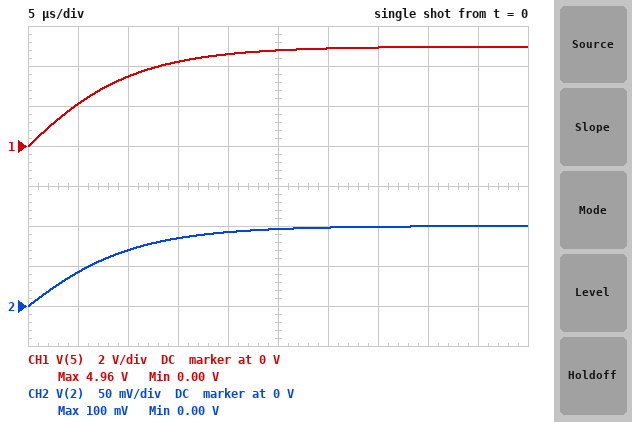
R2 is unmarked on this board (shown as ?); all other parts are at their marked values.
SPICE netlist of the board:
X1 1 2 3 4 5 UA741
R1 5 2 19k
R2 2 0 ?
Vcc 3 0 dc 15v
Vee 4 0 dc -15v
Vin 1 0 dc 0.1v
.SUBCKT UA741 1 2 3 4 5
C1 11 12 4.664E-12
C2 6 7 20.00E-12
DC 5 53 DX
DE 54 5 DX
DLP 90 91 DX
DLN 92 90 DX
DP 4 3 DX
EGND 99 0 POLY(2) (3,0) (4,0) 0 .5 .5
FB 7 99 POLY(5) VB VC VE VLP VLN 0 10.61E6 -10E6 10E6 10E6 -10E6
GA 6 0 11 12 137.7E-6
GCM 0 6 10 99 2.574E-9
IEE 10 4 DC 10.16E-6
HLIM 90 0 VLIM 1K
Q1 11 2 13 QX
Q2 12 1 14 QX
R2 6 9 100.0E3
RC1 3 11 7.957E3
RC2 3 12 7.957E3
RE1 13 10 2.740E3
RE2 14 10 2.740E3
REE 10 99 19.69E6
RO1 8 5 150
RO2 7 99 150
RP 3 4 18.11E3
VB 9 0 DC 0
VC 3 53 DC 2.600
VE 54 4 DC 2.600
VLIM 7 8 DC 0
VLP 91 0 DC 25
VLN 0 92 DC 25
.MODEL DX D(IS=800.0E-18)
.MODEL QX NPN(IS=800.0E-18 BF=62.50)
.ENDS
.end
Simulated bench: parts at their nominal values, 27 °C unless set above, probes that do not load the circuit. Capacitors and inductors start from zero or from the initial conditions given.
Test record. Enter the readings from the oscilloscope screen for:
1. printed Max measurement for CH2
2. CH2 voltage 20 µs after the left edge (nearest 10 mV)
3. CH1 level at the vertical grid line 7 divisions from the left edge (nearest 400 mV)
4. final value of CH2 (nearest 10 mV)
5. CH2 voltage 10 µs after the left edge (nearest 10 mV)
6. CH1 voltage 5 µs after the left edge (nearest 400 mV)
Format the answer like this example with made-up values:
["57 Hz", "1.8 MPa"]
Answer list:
["100 mV", "90 mV", "4.8 V", "100 mV", "70 mV", "2.0 V"]
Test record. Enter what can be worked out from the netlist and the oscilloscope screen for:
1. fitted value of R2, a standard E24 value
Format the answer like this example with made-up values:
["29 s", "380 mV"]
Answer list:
["390 Ω"]
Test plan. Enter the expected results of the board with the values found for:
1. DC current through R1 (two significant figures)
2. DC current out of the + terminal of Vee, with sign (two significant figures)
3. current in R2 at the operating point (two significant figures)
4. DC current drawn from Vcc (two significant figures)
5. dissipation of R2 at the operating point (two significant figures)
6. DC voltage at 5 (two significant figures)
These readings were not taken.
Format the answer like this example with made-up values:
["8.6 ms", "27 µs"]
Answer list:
["260 µA", "-1.7 mA", "260 µA", "1.7 mA", "26 µW", "5.0 V"]
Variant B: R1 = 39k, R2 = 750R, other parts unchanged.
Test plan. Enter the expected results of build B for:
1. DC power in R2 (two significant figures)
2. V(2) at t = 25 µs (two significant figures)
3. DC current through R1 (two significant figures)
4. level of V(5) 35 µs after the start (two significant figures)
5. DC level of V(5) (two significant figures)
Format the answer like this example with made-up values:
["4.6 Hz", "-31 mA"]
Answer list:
["13 µW", "95 mV", "130 µA", "5.2 V", "5.3 V"]
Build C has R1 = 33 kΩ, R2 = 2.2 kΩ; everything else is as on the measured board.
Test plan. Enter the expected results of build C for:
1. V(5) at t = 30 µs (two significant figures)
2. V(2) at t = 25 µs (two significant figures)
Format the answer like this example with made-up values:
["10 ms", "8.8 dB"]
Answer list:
["1.6 V", "100 mV"]
